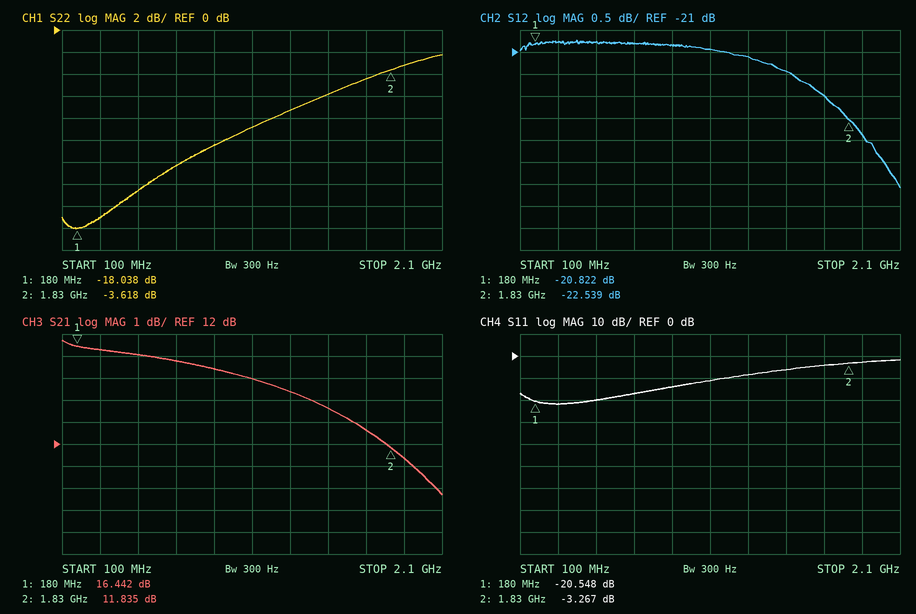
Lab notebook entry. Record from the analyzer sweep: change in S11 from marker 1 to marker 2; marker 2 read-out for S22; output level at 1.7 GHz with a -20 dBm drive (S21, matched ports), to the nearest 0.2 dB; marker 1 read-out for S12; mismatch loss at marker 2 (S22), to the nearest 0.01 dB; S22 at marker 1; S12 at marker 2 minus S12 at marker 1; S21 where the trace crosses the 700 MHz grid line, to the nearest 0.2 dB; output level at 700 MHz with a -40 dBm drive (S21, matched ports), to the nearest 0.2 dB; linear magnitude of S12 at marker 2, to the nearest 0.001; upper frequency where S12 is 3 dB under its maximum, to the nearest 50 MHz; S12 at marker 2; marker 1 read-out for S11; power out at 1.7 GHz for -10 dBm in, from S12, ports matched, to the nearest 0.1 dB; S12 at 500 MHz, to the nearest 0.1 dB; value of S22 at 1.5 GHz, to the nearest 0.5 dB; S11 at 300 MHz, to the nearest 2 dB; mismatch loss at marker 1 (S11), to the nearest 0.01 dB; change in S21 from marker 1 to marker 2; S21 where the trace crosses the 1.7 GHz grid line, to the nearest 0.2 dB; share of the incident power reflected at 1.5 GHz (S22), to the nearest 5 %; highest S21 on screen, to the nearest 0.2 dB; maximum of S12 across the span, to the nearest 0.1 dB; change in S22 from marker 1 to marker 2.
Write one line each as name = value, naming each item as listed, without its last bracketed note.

change in S11 from marker 1 to marker 2 = 17.281 dB
marker 2 read-out for S22 = -3.618 dB
output level at 1.7 GHz with a -20 dBm drive (S21, matched ports), to the nearest 0.2 dB = -7.4 dBm
marker 1 read-out for S12 = -20.822 dB
mismatch loss at marker 2 (S22), to the nearest 0.01 dB = 2.48 dB
S22 at marker 1 = -18.038 dB
S12 at marker 2 minus S12 at marker 1 = -1.717 dB
S21 where the trace crosses the 700 MHz grid line, to the nearest 0.2 dB = 15.8 dB
output level at 700 MHz with a -40 dBm drive (S21, matched ports), to the nearest 0.2 dB = -24.2 dBm
linear magnitude of S12 at marker 2, to the nearest 0.001 = 0.075
upper frequency where S12 is 3 dB under its maximum, to the nearest 50 MHz = 2.05 GHz
S12 at marker 2 = -22.539 dB
marker 1 read-out for S11 = -20.548 dB
power out at 1.7 GHz for -10 dBm in, from S12, ports matched, to the nearest 0.1 dB = -32.0 dBm
S12 at 500 MHz, to the nearest 0.1 dB = -20.8 dB
value of S22 at 1.5 GHz, to the nearest 0.5 dB = -6.0 dB
S11 at 300 MHz, to the nearest 2 dB = -22 dB
mismatch loss at marker 1 (S11), to the nearest 0.01 dB = 0.04 dB
change in S21 from marker 1 to marker 2 = -4.607 dB
S21 where the trace crosses the 1.7 GHz grid line, to the nearest 0.2 dB = 12.6 dB
share of the incident power reflected at 1.5 GHz (S22), to the nearest 5 % = 25 %
highest S21 on screen, to the nearest 0.2 dB = 16.8 dB
maximum of S12 across the span, to the nearest 0.1 dB = -20.7 dB
change in S22 from marker 1 to marker 2 = 14.420 dB
